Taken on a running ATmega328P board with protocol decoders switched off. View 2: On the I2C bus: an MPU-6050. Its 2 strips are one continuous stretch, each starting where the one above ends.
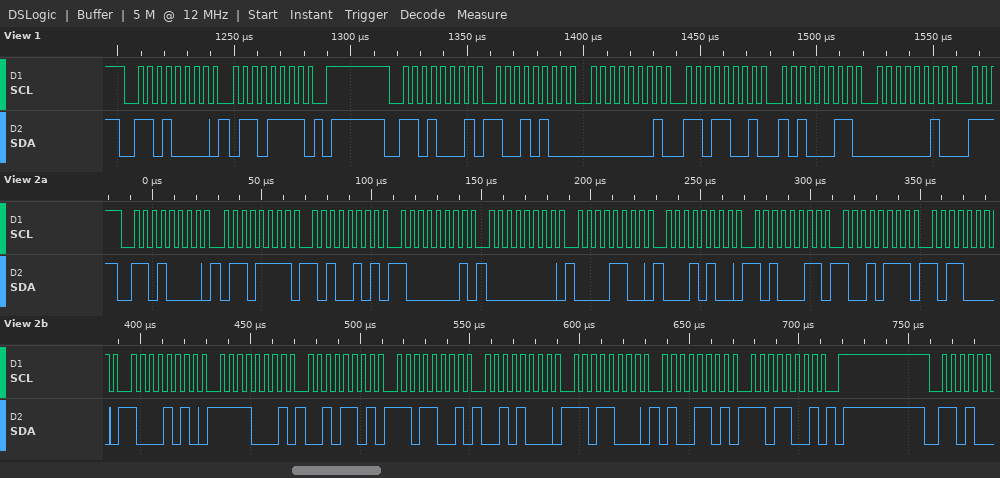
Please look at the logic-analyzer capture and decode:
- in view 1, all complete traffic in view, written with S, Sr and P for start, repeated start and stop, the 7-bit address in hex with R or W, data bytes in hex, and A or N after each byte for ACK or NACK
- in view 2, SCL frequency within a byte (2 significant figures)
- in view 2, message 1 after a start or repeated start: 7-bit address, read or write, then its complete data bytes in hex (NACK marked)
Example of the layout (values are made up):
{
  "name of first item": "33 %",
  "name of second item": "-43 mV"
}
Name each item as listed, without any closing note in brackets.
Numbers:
{
  "in view 1, all complete traffic in view, written with S, Sr and P for start, repeated start and stop, the 7-bit address in hex with R or W, data bytes in hex, and A or N after each byte for ACK or NACK": "S 68W A 6F A P S 68R A 94 A 01 A D9 A A3 A 02 A",
  "in view 2, SCL frequency within a byte": "250 kHz",
  "in view 2, message 1 after a start or repeated start: 7-bit address, read or write, then its complete data bytes in hex": "0x68 write: 6F A5 81 00 0C 14 A3 97 B0 8A F1 2D D9 28 D8 4D D9"
}
